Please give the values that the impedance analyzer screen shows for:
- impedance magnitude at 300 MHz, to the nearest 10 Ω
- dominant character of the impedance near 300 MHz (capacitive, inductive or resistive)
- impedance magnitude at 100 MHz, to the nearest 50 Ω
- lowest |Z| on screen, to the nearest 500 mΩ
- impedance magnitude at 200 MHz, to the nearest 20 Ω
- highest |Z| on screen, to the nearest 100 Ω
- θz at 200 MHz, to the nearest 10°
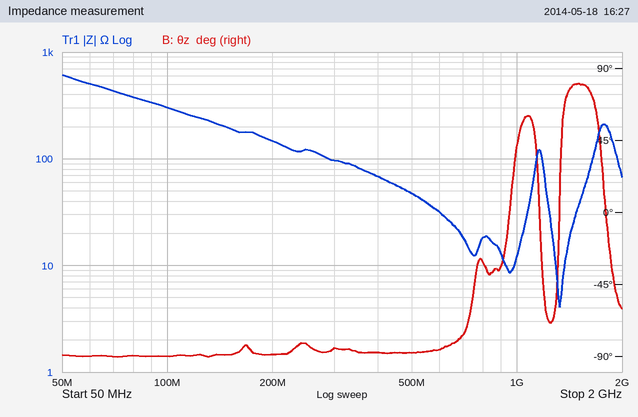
100 Ω
capacitive
300 Ω
4.0 Ω
140 Ω
600 Ω
-90°
